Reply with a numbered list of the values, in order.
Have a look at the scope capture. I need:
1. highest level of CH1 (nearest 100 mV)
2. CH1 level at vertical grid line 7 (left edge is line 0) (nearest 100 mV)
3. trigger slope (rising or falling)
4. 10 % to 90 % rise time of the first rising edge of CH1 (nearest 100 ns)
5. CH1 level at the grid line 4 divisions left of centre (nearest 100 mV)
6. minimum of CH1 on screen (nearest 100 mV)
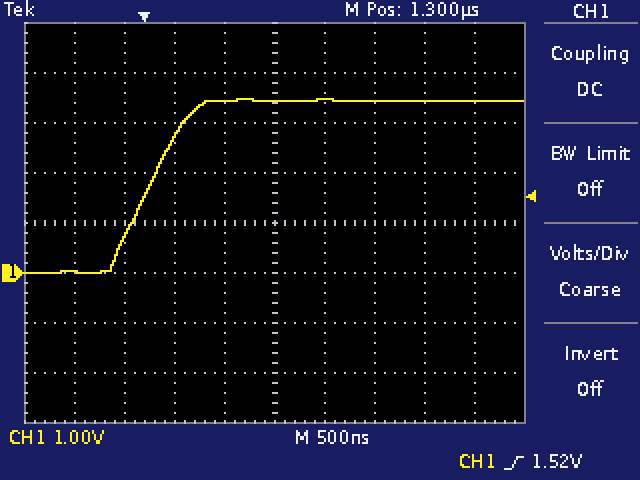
1. 3.5 V
2. 3.4 V
3. rising
4. 700 ns
5. 0.0 V
6. 0.0 V
